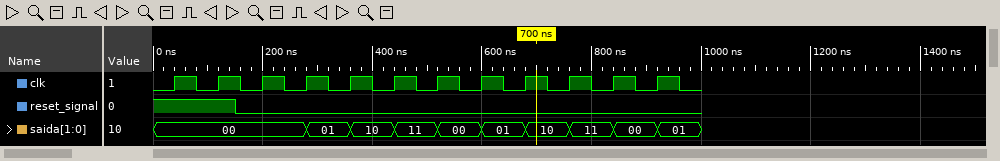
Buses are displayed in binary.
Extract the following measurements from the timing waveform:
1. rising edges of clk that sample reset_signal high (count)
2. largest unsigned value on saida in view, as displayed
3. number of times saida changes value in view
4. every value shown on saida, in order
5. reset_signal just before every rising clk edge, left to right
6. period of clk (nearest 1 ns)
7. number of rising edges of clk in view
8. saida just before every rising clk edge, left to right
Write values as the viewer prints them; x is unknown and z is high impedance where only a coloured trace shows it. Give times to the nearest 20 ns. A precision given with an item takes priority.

2
11
9
00, 01, 10, 11, 00, 01, 10, 11, 00, 01
1 1 0 0 0 0 0 0 0 0 0 0
80 ns
12
00, 00, 00, 00, 01, 10, 11, 00, 01, 10, 11, 00
